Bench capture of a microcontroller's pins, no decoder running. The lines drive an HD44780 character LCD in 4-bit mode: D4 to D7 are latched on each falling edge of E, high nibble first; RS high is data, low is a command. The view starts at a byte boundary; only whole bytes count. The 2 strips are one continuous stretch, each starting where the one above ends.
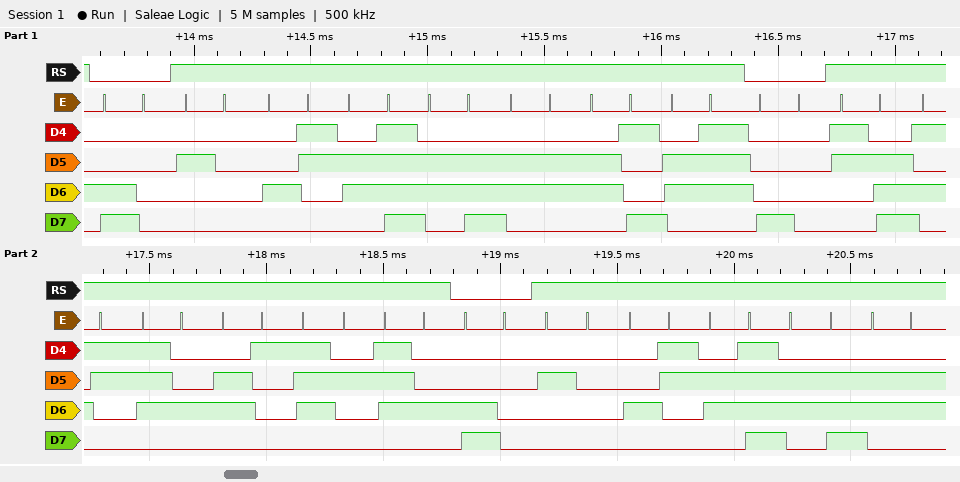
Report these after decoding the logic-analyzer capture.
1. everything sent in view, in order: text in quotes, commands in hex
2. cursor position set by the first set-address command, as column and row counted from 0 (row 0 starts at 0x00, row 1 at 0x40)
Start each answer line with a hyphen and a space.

- 0xC0 " Config" 0x80 ">Start" 0xC0 " Conf"
- column 0, row 1
